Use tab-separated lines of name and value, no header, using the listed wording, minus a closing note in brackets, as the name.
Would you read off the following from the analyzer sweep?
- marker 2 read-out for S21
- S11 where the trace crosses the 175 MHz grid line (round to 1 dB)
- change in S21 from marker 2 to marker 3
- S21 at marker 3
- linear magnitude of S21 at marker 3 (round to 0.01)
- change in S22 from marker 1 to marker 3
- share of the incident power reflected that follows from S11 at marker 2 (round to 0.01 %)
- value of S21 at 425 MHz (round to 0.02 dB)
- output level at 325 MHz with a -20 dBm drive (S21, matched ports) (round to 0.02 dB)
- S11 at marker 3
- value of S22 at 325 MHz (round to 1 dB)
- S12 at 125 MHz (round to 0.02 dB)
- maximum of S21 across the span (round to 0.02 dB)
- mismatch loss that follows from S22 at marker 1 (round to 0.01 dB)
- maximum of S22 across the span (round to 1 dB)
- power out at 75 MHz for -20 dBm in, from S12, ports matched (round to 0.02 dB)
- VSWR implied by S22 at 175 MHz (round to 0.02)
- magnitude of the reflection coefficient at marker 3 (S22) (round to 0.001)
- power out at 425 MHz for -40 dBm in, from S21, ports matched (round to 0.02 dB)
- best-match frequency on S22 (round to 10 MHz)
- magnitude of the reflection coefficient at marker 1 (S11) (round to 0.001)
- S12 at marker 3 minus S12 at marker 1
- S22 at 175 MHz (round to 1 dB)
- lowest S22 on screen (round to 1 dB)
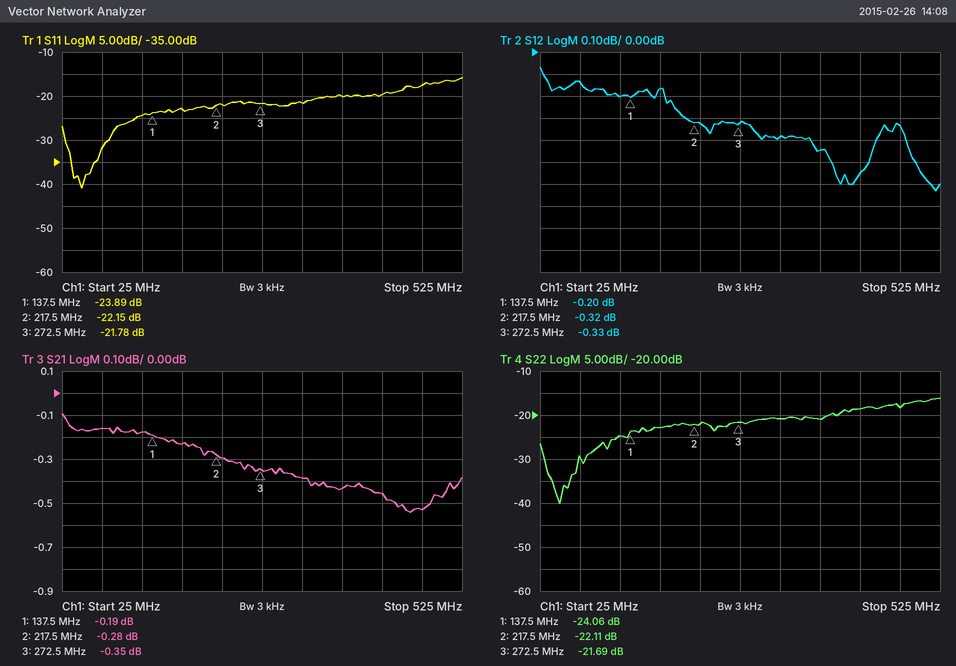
marker 2 read-out for S21	-0.28 dB
S11 where the trace crosses the 175 MHz grid line	-23 dB
change in S21 from marker 2 to marker 3	-0.07 dB
S21 at marker 3	-0.35 dB
linear magnitude of S21 at marker 3	0.96
change in S22 from marker 1 to marker 3	2.37 dB
share of the incident power reflected that follows from S11 at marker 2	0.61 %
value of S21 at 425 MHz	-0.46 dB
output level at 325 MHz with a -20 dBm drive (S21, matched ports)	-20.38 dBm
S11 at marker 3	-21.78 dB
value of S22 at 325 MHz	-21 dB
S12 at 125 MHz	-0.20 dB
maximum of S21 across the span	-0.10 dB
mismatch loss that follows from S22 at marker 1	0.02 dB
maximum of S22 across the span	-16 dB
power out at 75 MHz for -20 dBm in, from S12, ports matched	-20.14 dBm
VSWR implied by S22 at 175 MHz	1.16
magnitude of the reflection coefficient at marker 3 (S22)	0.082
power out at 425 MHz for -40 dBm in, from S21, ports matched	-40.46 dBm
best-match frequency on S22	50 MHz
magnitude of the reflection coefficient at marker 1 (S11)	0.064
S12 at marker 3 minus S12 at marker 1	-0.13 dB
S22 at 175 MHz	-23 dB
lowest S22 on screen	-40 dB
